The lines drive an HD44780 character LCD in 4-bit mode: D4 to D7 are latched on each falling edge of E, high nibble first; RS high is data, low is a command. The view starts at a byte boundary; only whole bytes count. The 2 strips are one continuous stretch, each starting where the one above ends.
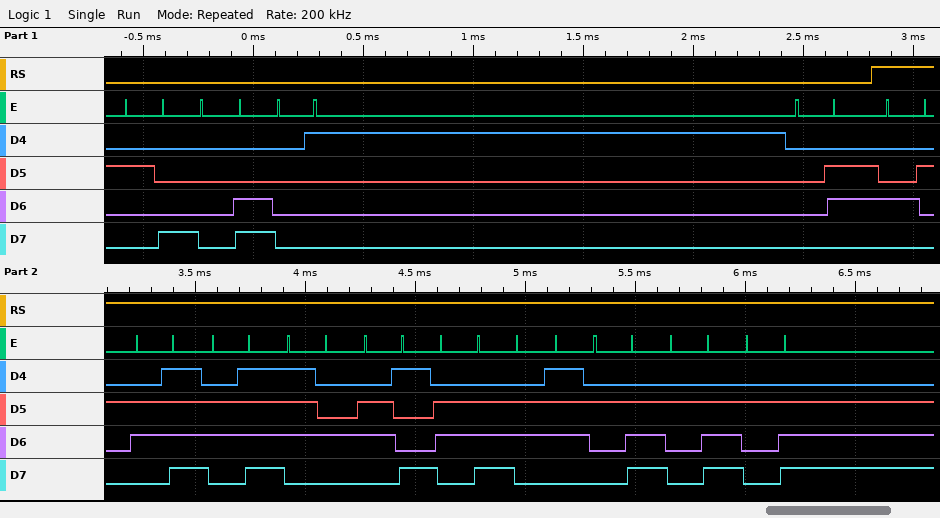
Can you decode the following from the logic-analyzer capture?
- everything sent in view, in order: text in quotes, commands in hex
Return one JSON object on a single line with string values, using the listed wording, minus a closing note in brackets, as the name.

{"everything sent in view, in order: text in quotes, commands in hex": "0x28 0x0C 0x01 0x06 \"Booting...\""}
